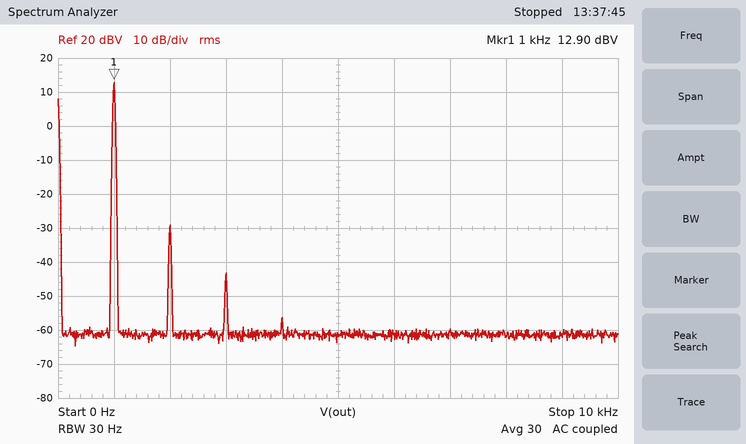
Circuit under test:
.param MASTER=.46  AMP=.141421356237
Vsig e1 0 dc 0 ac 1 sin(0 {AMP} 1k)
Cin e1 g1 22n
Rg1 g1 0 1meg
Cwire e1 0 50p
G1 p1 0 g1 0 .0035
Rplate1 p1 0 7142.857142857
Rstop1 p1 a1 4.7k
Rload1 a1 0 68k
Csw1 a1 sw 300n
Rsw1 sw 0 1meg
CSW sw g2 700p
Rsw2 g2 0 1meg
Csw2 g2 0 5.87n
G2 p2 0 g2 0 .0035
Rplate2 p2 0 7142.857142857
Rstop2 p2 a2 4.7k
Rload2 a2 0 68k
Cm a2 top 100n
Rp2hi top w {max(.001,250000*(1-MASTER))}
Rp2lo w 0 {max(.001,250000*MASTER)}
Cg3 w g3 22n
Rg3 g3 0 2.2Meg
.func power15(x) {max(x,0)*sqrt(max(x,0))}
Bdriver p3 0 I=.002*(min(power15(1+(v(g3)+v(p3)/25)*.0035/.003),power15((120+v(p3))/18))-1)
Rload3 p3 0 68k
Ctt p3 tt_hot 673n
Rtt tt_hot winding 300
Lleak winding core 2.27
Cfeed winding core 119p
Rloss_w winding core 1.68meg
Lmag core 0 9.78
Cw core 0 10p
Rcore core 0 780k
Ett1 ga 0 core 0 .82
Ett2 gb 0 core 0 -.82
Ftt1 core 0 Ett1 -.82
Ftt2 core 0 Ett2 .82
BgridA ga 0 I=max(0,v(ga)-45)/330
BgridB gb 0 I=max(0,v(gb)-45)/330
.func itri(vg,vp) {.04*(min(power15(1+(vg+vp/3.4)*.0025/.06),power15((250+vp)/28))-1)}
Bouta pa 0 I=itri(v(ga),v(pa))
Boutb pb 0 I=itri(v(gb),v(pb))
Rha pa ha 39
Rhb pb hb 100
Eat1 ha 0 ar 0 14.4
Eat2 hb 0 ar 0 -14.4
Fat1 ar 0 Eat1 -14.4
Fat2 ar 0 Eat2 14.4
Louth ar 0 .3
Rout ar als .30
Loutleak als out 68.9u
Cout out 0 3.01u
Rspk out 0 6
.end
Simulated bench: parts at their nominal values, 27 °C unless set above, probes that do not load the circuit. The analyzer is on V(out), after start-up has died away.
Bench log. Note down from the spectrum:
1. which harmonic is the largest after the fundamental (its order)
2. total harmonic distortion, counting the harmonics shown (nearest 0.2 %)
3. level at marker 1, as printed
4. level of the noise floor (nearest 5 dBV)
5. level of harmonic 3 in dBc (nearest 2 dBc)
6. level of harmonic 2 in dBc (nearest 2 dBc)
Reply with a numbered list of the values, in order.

1. 2
2. 0.8 %
3. 12.90 dBV
4. -60 dBV
5. -56 dBc
6. -42 dBc
